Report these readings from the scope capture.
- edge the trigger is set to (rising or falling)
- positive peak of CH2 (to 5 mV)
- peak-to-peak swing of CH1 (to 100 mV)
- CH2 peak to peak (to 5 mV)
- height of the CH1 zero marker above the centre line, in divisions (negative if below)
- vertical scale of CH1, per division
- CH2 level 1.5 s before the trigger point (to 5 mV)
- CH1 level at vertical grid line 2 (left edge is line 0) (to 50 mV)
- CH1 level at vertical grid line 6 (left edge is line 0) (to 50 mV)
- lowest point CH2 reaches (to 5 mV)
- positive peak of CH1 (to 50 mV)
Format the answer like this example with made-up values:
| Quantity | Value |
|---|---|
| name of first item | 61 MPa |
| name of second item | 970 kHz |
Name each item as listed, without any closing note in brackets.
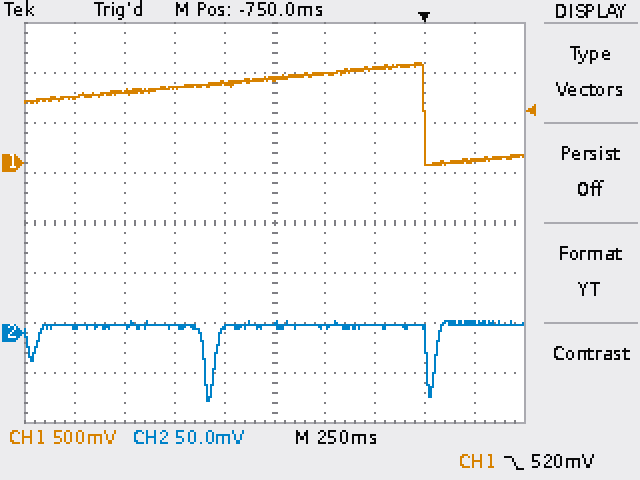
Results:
| Quantity | Value |
|---|---|
| edge the trigger is set to | falling |
| positive peak of CH2 | 10 mV |
| peak-to-peak swing of CH1 | 1.00 V |
| CH2 peak to peak | 80 mV |
| height of the CH1 zero marker above the centre line, in divisions | +1.2 div |
| vertical scale of CH1, per division | 500 mV |
| CH2 level 1.5 s before the trigger point | 5 mV |
| CH1 level at vertical grid line 2 (left edge is line 0) | 700 mV |
| CH1 level at vertical grid line 6 (left edge is line 0) | 900 mV |
| lowest point CH2 reaches | -70 mV |
| positive peak of CH1 | 1.00 V |
